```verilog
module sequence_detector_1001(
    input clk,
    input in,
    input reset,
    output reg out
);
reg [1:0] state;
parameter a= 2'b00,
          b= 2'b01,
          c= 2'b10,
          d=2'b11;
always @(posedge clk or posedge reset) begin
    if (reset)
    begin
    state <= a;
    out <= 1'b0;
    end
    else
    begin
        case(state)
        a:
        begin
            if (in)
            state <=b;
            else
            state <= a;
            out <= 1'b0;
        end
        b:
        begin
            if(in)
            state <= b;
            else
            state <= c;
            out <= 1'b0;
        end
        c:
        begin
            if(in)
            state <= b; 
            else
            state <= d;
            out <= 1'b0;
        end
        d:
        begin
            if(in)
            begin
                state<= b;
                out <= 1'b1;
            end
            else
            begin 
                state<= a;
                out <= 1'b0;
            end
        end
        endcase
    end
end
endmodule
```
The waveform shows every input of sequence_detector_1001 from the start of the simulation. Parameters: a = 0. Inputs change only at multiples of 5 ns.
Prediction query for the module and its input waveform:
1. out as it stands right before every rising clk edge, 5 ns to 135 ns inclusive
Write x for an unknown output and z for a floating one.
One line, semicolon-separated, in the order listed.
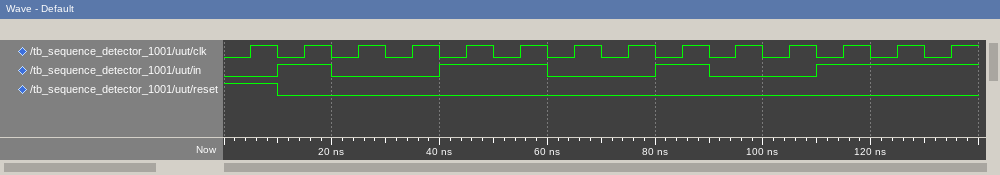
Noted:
0 0 0 0 0 1 0 0 0 1 0 0 1 0
